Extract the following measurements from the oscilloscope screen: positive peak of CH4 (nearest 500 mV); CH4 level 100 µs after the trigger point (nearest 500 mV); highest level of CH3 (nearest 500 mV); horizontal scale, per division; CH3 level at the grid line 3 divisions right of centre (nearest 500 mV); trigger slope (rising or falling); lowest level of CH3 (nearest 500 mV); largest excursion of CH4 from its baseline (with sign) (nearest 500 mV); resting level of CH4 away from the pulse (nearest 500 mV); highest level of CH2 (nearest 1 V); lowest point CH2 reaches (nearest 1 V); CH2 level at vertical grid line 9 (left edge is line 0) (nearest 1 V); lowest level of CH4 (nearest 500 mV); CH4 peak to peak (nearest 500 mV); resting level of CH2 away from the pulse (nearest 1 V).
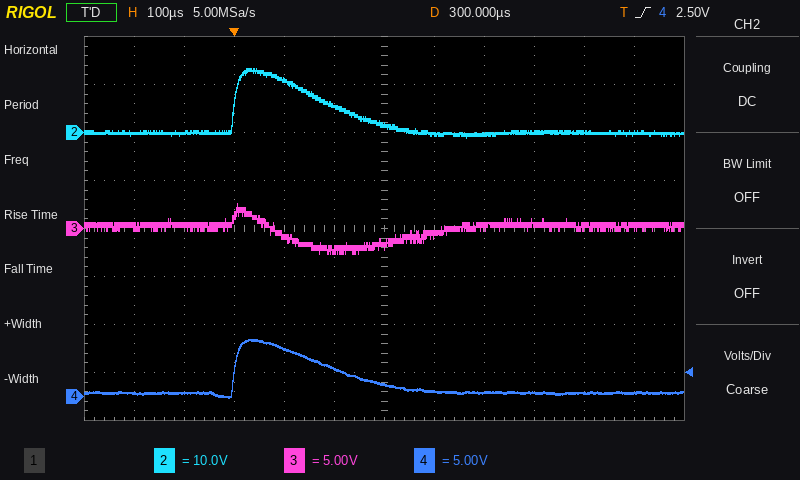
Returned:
6.0 V
5.0 V
2.5 V
100 µs
500 mV
rising
-2.5 V
+5.5 V
500 mV
13 V
-1 V
0 V
0.0 V
6.0 V
0 V
